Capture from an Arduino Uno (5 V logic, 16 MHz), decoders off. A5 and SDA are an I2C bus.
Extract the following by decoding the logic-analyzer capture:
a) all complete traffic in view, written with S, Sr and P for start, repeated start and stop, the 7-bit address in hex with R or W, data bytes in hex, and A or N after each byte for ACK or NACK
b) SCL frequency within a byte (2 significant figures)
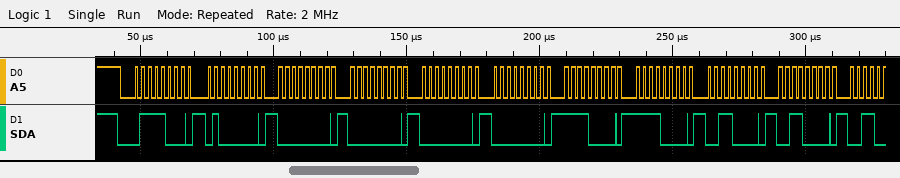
S 3CW A 40 A 00 A 00 A 00 A 00 A F0 A F0 A 30 A 30 A
400 kHz
